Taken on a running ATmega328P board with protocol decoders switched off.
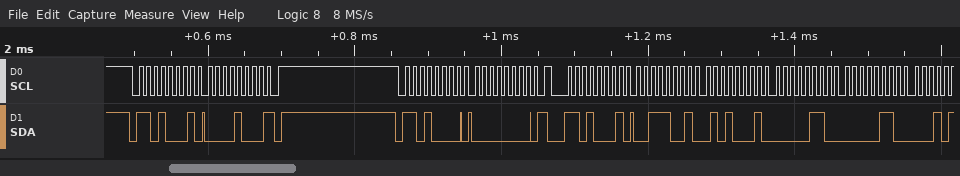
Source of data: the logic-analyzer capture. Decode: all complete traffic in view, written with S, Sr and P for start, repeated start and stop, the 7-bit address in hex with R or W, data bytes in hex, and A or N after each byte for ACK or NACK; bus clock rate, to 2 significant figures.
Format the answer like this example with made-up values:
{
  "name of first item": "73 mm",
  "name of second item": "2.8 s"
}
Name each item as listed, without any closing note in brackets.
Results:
{
  "all complete traffic in view, written with S, Sr and P for start, repeated start and stop, the 7-bit address in hex with R or W, data bytes in hex, and A or N after each byte for ACK or NACK": "S 68R A 08 N P S 68W A 00 A Sr 68R A 39 A 51 A 06 A 06 A",
  "bus clock rate, to 2 significant figures": "100 kHz"
}
